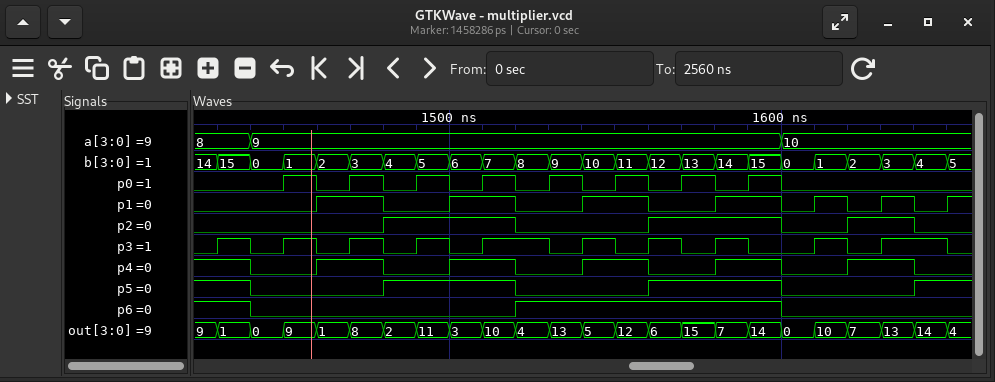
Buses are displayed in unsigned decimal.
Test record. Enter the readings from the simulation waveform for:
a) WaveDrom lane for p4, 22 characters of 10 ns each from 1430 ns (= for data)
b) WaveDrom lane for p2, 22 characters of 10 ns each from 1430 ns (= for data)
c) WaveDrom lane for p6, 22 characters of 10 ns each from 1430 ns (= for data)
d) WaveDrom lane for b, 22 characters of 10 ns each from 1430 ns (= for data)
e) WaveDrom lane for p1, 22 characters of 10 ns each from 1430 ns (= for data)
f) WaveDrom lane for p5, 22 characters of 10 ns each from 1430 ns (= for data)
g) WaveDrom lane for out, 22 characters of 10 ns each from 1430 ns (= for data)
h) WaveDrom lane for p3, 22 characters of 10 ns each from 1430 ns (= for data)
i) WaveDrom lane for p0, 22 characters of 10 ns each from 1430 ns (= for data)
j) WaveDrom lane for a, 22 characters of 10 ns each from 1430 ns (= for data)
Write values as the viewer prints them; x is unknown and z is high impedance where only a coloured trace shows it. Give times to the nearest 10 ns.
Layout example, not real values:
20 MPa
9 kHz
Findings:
{name: 'p4', wave: '10.1.0.1.0.1.0.1.0.1.0'}
{name: 'p2', wave: '0....1...0...1...0.1.0'}
{name: 'p6', wave: '10.......1.......0....'}
{name: 'b', wave: '======================', data: '15 0 1 2 3 4 5 6 7 8 9 10 11 12 13 14 15 0 1 2 3 4'}
{name: 'p1', wave: '0..1.0.1.0.1.0.1.01010'}
{name: 'p5', wave: '10...1...0...1...0...1'}
{name: 'out', wave: '======================', data: '1 0 9 1 8 2 11 3 10 4 13 5 12 6 15 7 14 0 10 7 13 14'}
{name: 'p3', wave: '101010101.0101010.101.'}
{name: 'p0', wave: '0.1010101010101010....'}
{name: 'a', wave: '==...............=....', data: '8 9 10'}
